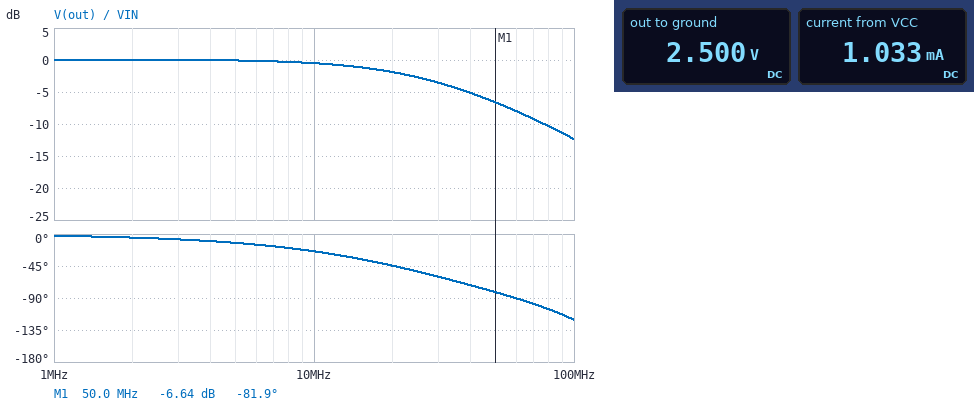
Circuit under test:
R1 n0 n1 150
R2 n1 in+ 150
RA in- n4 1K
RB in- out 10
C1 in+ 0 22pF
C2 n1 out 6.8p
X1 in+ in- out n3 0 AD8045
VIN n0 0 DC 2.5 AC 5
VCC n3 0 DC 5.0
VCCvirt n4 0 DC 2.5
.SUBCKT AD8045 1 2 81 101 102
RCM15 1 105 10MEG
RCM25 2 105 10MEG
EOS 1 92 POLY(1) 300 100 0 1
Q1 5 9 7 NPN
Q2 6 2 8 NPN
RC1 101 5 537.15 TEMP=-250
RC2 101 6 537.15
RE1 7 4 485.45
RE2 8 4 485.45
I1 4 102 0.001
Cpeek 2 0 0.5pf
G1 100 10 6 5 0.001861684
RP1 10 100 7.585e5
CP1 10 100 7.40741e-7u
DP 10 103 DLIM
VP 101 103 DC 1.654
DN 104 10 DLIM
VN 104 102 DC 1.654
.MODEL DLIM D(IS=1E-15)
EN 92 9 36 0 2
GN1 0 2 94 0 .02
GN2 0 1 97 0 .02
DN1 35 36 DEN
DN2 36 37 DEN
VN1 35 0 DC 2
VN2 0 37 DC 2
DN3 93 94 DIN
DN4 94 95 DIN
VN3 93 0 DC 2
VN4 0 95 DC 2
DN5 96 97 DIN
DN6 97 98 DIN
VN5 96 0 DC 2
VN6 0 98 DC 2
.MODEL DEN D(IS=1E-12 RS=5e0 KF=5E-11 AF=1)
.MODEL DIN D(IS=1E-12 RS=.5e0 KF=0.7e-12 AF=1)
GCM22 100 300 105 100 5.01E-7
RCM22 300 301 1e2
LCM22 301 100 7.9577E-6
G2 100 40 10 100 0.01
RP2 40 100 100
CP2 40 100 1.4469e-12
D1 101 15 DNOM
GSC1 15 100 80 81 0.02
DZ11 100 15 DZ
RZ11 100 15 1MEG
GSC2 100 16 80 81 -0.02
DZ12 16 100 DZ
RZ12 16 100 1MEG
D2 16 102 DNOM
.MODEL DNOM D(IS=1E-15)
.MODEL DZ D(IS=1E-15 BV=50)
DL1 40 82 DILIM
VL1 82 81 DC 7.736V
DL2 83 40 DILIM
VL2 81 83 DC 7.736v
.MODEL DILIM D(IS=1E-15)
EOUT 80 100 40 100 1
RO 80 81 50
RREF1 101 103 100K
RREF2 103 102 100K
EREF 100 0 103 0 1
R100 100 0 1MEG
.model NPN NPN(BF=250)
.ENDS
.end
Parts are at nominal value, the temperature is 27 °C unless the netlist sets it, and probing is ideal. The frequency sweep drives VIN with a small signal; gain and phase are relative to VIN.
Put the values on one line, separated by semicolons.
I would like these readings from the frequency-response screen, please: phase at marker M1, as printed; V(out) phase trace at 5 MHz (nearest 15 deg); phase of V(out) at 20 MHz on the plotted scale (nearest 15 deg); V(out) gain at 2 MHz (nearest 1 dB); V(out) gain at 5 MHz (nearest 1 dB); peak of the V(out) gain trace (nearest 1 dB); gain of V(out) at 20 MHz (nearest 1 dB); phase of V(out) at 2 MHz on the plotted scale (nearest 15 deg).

-81.9 deg; -15 deg; -45 deg; 0 dB; 0 dB; 0 dB; -2 dB; 0 deg
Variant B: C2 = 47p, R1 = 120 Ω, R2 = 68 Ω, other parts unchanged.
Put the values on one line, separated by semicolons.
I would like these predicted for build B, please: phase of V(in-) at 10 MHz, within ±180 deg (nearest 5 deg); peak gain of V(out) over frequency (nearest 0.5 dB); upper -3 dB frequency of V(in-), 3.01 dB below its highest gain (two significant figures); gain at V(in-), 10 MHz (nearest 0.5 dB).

-15 deg; 0.5 dB; 51 MHz; 0 dB
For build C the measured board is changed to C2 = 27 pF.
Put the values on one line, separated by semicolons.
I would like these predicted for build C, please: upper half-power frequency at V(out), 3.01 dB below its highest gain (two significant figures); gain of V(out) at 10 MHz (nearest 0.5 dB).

33 MHz; 0 dB
